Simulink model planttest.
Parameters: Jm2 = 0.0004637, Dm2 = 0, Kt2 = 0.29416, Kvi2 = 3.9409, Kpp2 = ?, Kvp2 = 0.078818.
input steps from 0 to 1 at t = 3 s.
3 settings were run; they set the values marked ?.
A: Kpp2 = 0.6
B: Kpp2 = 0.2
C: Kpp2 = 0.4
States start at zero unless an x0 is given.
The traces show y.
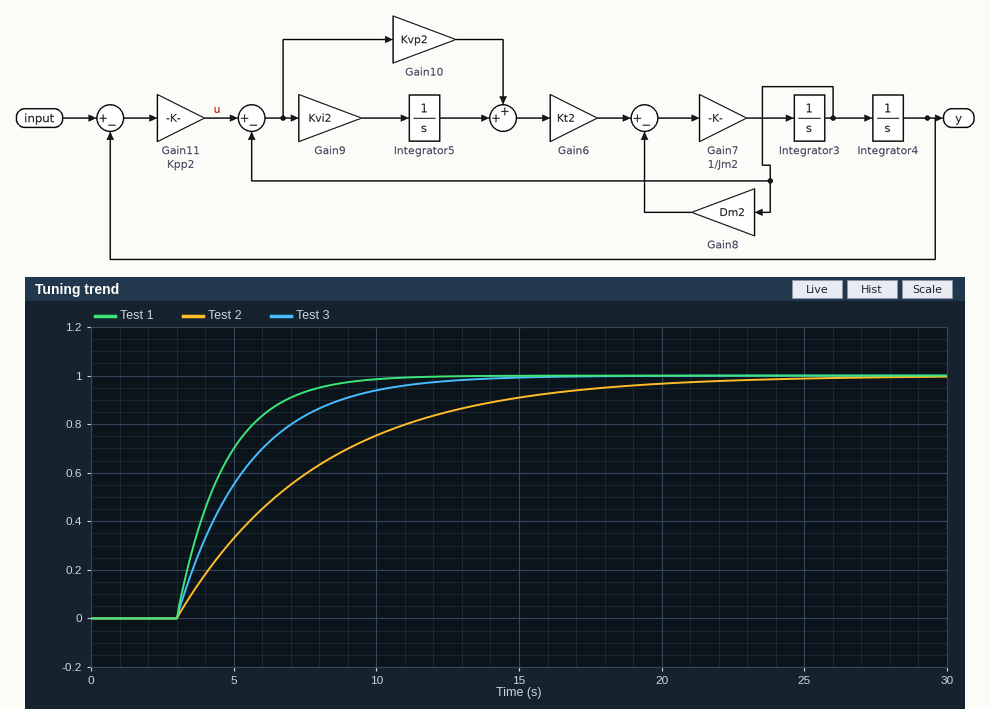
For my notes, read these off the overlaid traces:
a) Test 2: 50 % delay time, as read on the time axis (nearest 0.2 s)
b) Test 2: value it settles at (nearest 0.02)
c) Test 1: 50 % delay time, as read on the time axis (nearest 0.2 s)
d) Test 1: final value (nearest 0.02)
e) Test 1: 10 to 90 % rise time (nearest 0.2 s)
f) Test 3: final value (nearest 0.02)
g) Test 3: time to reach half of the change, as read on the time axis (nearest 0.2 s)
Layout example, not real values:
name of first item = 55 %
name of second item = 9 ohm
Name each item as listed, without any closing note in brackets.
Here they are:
Test 2: 50 % delay time, as read on the time axis = 6.4 s
Test 2: value it settles at = 1.00
Test 1: 50 % delay time, as read on the time axis = 4.2 s
Test 1: final value = 1.00
Test 1: 10 to 90 % rise time = 3.6 s
Test 3: final value = 1.00
Test 3: time to reach half of the change, as read on the time axis = 4.8 s
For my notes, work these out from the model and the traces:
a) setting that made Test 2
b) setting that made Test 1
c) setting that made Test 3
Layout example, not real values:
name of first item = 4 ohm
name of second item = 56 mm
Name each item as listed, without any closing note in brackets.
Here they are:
setting that made Test 2 = B
setting that made Test 1 = A
setting that made Test 3 = C
